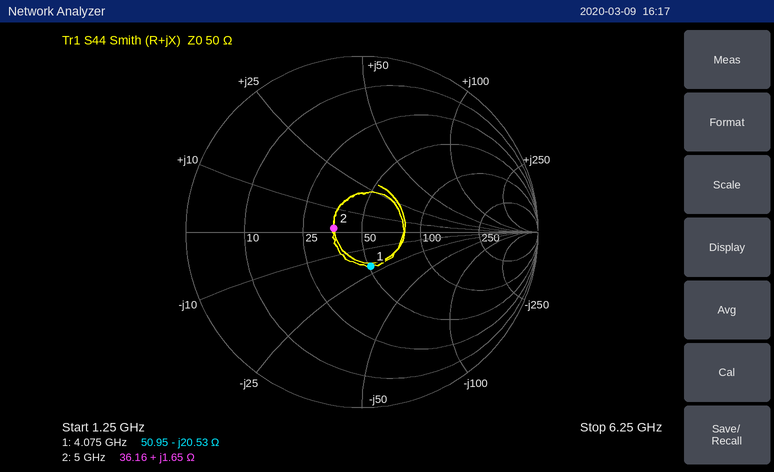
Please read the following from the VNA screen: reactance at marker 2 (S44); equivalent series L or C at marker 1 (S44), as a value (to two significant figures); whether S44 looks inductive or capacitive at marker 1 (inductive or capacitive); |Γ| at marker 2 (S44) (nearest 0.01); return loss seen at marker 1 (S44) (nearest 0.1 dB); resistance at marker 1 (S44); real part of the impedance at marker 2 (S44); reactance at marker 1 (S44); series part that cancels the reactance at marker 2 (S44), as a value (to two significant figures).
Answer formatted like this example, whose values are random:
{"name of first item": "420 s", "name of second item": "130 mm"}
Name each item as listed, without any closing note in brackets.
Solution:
{"reactance at marker 2": "+1.65 Ω", "equivalent series L or C at marker 1 (S44), as a value": "1.9 pF", "whether S44 looks inductive or capacitive at marker 1": "capacitive", "|Γ| at marker 2 (S44)": "0.16", "return loss seen at marker 1 (S44)": "14.0 dB", "resistance at marker 1": "50.95 Ω", "real part of the impedance at marker 2": "36.16 Ω", "reactance at marker 1": "-20.53 Ω", "series part that cancels the reactance at marker 2 (S44), as a value": "19 pF"}
